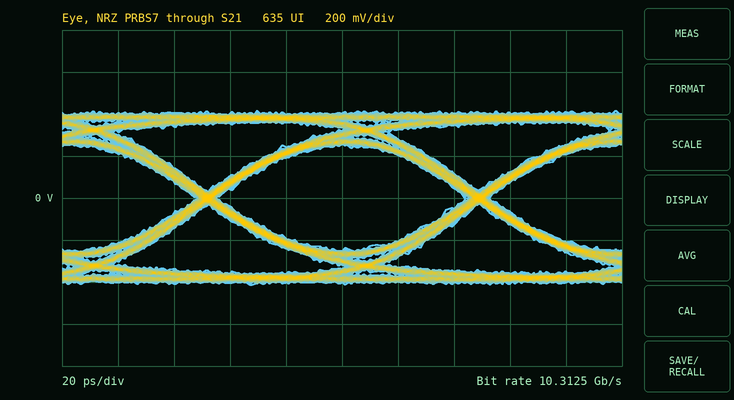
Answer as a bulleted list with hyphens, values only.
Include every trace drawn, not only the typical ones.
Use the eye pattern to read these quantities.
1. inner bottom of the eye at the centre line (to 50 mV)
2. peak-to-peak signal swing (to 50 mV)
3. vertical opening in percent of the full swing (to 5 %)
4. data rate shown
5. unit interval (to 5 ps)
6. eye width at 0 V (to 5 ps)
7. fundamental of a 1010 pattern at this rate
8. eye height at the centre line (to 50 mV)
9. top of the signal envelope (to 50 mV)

- -250 mV
- 850 mV
- 60 %
- 10.3125 Gb/s
- 95 ps
- 90 ps
- 5.15625 GHz
- 500 mV
- 400 mV
